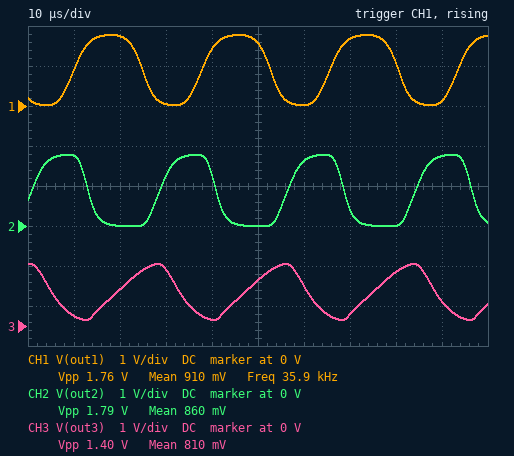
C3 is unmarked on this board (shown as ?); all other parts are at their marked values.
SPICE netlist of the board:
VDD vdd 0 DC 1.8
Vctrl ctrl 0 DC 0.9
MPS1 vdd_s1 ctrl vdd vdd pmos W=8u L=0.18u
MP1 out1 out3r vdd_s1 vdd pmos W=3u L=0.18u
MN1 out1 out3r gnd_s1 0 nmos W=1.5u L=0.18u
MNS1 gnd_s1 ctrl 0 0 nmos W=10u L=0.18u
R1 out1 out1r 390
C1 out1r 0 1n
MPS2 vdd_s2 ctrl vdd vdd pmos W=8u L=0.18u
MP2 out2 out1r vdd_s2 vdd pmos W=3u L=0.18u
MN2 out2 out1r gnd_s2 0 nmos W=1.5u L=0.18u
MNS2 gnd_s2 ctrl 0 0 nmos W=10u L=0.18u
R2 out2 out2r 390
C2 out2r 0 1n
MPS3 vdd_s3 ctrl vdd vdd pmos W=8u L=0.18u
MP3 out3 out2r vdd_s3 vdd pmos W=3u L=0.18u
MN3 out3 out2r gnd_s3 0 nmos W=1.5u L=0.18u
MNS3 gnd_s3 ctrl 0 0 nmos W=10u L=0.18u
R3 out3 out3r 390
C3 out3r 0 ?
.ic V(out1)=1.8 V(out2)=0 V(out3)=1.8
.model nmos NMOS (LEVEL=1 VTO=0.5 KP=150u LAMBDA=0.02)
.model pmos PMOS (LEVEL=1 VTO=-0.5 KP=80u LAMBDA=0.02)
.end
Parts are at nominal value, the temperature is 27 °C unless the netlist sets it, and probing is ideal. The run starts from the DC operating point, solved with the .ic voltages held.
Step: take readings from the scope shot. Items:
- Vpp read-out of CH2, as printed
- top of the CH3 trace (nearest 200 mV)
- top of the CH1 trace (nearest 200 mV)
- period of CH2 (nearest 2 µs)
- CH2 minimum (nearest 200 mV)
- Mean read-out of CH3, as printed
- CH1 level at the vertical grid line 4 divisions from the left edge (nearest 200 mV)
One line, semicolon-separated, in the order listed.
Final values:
1.79 V; 1.6 V; 1.8 V; 28 µs; 0 V; 810 mV; 1.4 V
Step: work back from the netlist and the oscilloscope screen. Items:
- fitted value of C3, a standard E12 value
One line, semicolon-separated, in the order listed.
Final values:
2.7 nF
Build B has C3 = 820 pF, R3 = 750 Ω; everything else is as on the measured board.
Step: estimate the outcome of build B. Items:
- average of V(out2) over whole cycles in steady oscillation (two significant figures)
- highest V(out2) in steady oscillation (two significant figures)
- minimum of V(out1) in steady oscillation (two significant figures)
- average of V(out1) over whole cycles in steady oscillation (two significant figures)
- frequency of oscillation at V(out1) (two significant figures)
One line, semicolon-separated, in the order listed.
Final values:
880 mV; 1.7 V; 19 mV; 840 mV; 54 kHz
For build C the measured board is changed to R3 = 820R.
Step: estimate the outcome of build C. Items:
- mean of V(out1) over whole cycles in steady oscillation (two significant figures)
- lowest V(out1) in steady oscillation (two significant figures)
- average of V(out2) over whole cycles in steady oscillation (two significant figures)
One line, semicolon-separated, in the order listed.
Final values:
930 mV; 18 mV; 800 mV
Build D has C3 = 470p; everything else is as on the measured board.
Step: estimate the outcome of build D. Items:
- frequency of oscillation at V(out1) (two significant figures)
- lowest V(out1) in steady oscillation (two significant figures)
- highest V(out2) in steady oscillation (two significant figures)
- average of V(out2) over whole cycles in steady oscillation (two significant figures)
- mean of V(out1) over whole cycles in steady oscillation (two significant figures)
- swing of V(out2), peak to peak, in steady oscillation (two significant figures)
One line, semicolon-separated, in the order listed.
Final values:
64 kHz; 28 mV; 1.7 V; 910 mV; 810 mV; 1.6 V
